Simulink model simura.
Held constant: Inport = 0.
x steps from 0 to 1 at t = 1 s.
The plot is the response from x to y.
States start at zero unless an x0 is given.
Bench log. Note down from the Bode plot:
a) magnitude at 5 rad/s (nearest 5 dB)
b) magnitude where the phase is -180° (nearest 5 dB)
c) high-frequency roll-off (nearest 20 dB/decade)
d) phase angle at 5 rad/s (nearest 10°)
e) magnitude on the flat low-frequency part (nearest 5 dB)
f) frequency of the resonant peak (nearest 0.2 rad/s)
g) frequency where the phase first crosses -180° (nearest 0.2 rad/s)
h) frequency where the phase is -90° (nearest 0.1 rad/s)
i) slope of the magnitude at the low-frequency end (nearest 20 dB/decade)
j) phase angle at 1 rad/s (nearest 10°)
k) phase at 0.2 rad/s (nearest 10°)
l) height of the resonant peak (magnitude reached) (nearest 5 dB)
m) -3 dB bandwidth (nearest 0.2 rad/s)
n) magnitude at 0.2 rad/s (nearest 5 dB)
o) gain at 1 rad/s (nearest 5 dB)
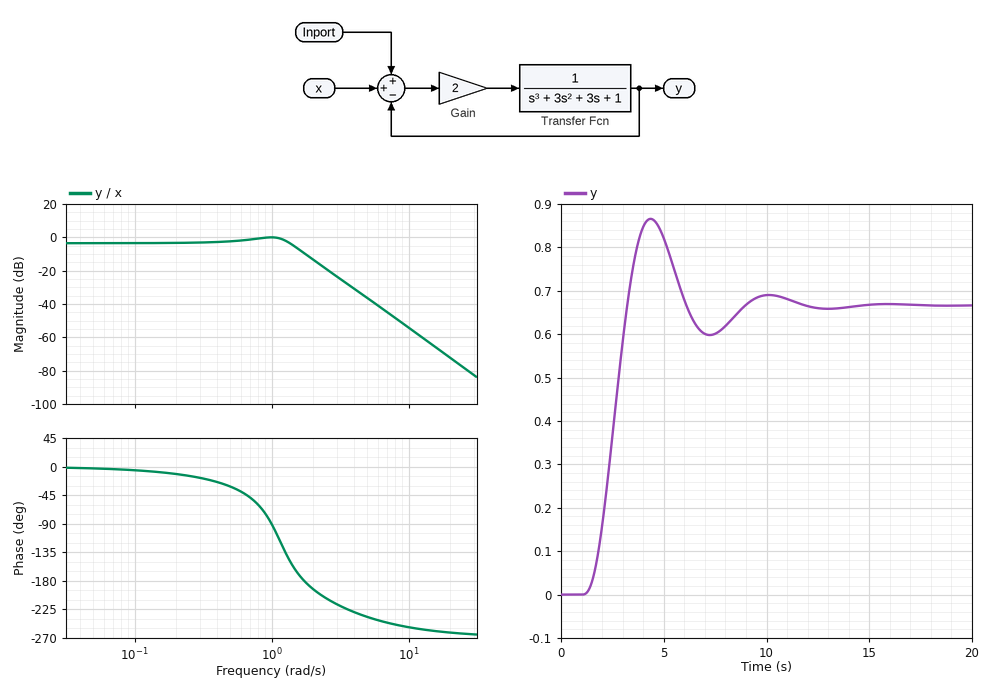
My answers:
-35 dB
-10 dB
-60 dB/decade
-240°
-5 dB
1.0 rad/s
1.8 rad/s
1.0 rad/s
0 dB/decade
-90°
-10°
0 dB
1.6 rad/s
-5 dB
0 dB
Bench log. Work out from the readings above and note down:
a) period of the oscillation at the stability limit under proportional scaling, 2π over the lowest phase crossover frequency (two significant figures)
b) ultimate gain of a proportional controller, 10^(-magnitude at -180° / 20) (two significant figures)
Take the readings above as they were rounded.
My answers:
3.5 s
3.2
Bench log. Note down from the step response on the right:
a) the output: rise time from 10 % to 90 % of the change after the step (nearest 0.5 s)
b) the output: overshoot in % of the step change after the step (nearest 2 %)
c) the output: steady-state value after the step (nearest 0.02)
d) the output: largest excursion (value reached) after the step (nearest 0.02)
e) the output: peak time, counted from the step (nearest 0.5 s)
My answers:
1.5 s
30 %
0.66
0.86
3.5 s
